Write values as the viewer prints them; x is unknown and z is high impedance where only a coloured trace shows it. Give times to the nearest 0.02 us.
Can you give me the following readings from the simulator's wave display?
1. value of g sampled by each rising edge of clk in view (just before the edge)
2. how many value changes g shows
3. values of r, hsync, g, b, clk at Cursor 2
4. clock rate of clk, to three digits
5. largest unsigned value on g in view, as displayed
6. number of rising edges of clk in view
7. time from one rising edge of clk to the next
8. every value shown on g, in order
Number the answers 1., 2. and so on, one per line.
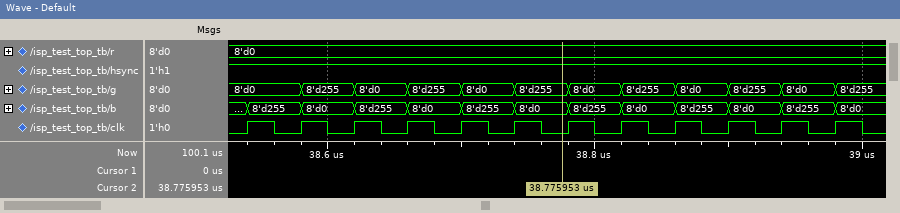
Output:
1. 8'd0, 8'd0, 8'd255, 8'd0, 8'd255, 8'd0, 8'd255, 8'd0, 8'd255, 8'd0, 8'd255, 8'd0
2. 11
3. r=8'd0, hsync=1, g=8'd255, b=8'd0, clk=0
4. 25.0 MHz
5. 8'd255
6. 12
7. 0.04 us
8. 8'd0, 8'd255, 8'd0, 8'd255, 8'd0, 8'd255, 8'd0, 8'd255, 8'd0, 8'd255, 8'd0, 8'd255
